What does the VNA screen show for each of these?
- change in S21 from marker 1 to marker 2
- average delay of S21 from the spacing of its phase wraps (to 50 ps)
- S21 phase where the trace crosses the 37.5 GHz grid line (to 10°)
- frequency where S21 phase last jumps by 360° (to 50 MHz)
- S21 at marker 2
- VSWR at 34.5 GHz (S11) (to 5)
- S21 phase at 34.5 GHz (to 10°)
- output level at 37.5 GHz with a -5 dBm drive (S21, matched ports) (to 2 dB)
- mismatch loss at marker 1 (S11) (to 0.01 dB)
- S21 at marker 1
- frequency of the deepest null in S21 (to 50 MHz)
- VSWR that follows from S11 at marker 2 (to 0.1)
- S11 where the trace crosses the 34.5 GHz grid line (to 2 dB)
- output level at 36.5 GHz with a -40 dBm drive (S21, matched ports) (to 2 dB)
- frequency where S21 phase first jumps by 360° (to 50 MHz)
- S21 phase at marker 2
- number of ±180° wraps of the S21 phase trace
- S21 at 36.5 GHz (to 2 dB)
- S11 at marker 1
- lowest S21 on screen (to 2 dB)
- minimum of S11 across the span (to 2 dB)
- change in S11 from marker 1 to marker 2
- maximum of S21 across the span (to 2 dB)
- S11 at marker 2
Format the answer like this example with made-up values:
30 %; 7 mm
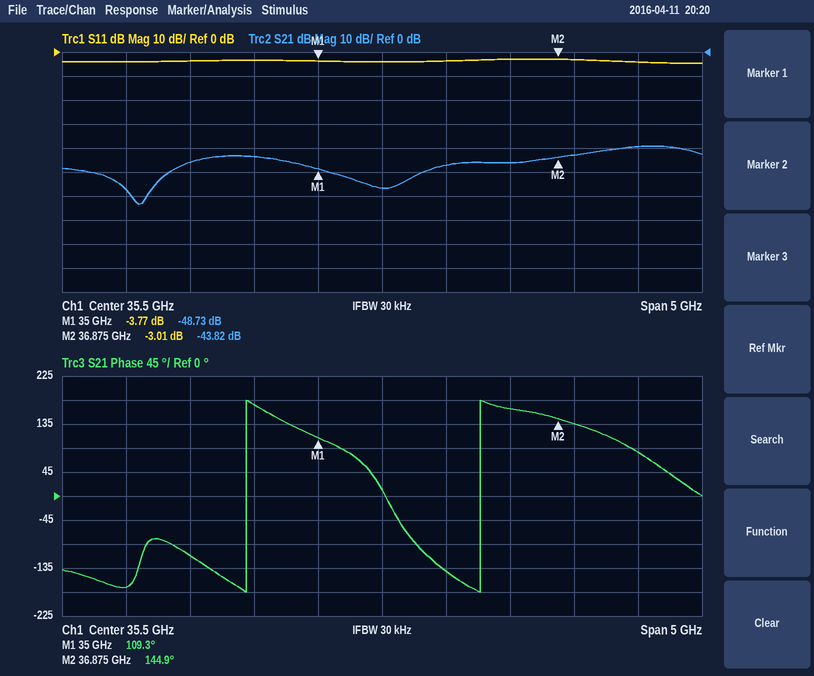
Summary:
4.91 dB; 550 ps; 80°; 36.25 GHz; -43.82 dB; 5; 170°; -44 dBm; 2.36 dB; -48.73 dB; 33.60 GHz; 5.8; -4 dB; -86 dBm; 34.45 GHz; 144.9°; 2; -46 dB; -3.77 dB; -64 dB; -4 dB; 0.76 dB; -40 dB; -3.01 dB
